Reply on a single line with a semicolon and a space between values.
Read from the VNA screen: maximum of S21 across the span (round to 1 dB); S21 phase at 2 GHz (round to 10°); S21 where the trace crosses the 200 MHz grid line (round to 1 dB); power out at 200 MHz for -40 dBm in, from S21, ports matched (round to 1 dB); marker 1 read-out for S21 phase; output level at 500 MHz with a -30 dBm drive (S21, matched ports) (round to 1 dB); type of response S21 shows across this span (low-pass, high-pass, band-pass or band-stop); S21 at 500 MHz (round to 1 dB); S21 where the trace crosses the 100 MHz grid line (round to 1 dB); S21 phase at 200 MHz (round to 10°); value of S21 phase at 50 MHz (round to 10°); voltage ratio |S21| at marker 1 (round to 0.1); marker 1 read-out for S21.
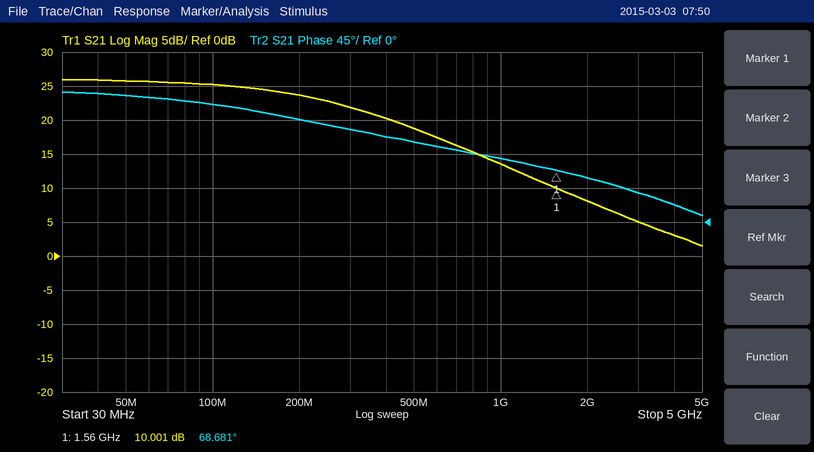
26 dB; 60°; 24 dB; -16 dBm; 68.681°; -11 dBm; low-pass; 19 dB; 25 dB; 140°; 170°; 3.2; 10.001 dB
